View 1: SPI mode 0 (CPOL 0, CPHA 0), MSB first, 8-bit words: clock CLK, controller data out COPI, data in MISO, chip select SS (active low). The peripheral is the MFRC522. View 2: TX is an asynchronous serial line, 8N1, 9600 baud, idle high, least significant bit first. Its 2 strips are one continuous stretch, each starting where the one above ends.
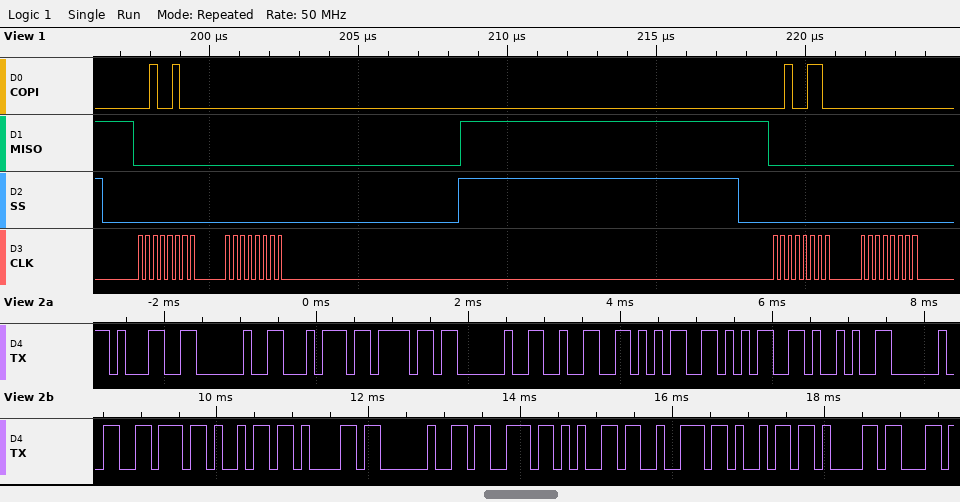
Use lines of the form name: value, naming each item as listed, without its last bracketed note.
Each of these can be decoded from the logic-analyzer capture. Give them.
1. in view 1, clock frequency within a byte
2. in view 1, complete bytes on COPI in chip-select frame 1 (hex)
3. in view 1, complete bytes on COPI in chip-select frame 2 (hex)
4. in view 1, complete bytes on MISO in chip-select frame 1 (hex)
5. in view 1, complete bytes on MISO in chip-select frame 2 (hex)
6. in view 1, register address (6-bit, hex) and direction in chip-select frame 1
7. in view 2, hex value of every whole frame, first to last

in view 1, clock frequency within a byte: 4 MHz
in view 1, complete bytes on COPI in chip-select frame 1: 24 00
in view 1, complete bytes on COPI in chip-select frame 2: 26 00
in view 1, complete bytes on MISO in chip-select frame 1: 00 00
in view 1, complete bytes on MISO in chip-select frame 2: 00 00
in view 1, register address (6-bit, hex) and direction in chip-select frame 1: 0x12 write
in view 2, hex value of every whole frame, first to last: 31 20 74 6F 20 32 35 35 29 20 76 69 61 20 73 65 72 69 61
